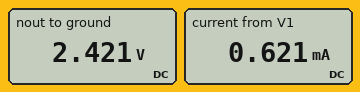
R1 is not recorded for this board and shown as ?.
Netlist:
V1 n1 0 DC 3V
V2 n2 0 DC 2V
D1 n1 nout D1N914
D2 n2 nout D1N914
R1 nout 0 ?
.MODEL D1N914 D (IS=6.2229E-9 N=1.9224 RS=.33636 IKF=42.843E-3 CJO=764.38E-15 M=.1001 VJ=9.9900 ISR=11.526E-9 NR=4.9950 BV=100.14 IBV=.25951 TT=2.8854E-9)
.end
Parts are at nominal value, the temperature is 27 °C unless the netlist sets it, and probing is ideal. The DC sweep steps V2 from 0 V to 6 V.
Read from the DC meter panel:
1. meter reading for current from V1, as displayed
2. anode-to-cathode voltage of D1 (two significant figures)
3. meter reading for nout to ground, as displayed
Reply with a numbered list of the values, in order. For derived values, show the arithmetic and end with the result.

1. 0.621 mA
2. 3 V - 2.421 V = 580 mV
3. 2.421 V
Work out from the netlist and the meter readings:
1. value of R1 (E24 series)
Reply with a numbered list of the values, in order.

1. 3.9 kΩ
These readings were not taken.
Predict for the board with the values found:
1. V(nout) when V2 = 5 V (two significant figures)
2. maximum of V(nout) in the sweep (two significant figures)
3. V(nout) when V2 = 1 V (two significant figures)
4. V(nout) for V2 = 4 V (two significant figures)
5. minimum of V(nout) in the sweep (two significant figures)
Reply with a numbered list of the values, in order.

1. 4.4 V
2. 5.4 V
3. 2.4 V
4. 3.4 V
5. 2.4 V
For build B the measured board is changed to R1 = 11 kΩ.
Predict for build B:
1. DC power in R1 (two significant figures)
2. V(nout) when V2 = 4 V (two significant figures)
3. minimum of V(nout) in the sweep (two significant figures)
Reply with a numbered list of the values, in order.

1. 560 µW
2. 3.5 V
3. 2.5 V
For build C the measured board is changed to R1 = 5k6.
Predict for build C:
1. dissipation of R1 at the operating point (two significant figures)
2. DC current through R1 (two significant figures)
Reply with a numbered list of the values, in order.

1. 1.1 mW
2. 440 µA
